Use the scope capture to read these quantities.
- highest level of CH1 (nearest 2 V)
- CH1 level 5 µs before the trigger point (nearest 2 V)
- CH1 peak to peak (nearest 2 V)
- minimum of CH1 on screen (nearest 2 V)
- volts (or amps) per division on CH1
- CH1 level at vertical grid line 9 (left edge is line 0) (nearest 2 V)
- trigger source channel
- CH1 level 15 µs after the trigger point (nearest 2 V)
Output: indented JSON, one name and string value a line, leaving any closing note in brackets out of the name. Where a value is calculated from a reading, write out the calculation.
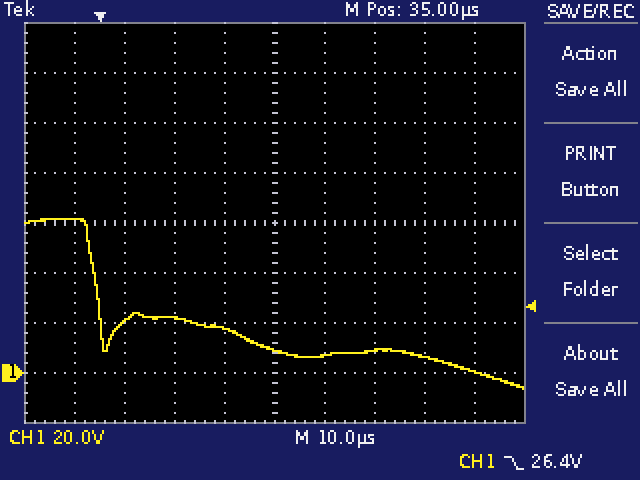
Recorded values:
{
  "highest level of CH1": "62 V",
  "CH1 level 5 µs before the trigger point": "62 V",
  "CH1 peak to peak": "62 V − (-6 V) = 68 V",
  "minimum of CH1 on screen": "-6 V",
  "volts (or amps) per division on CH1": "20 V",
  "CH1 level at vertical grid line 9 (left edge is line 0)": "0 V",
  "trigger source channel": "CH1",
  "CH1 level 15 µs after the trigger point": "22 V"
}
